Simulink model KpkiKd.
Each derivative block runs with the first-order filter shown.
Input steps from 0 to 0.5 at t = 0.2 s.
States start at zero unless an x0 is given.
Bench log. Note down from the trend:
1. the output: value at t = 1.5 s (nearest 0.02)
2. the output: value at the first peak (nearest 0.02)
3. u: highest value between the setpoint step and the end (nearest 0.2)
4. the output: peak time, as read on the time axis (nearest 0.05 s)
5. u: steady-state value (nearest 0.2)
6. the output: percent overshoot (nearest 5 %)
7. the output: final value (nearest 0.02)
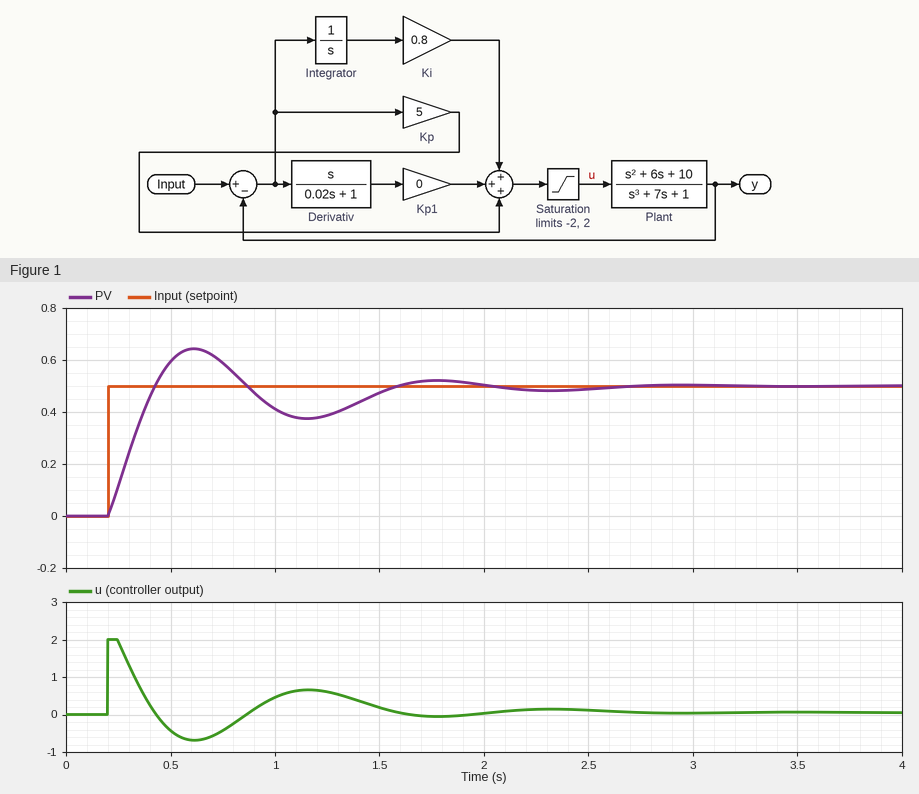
0.48
0.64
2.0
0.60 s
0.0
30 %
0.50
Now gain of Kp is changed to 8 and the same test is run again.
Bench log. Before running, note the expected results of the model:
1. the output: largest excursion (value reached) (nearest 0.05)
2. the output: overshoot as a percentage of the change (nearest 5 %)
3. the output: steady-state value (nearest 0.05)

0.60
25 %
0.50
